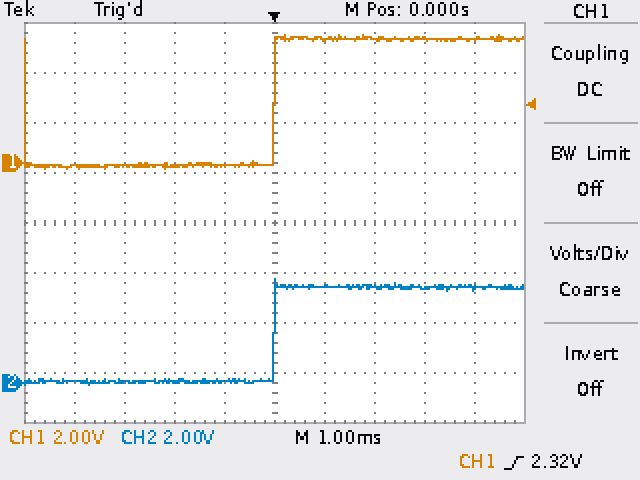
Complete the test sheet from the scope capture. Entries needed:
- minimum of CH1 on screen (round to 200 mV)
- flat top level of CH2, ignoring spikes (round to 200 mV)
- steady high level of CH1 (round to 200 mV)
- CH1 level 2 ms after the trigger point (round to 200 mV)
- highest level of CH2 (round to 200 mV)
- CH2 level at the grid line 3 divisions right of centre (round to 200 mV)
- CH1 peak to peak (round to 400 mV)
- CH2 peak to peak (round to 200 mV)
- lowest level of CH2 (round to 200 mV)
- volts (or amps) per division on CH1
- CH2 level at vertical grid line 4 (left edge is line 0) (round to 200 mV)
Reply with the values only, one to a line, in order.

-200 mV
3.8 V
5.0 V
5.0 V
4.2 V
3.8 V
5.2 V
4.2 V
0.0 V
2 V
0.0 V
